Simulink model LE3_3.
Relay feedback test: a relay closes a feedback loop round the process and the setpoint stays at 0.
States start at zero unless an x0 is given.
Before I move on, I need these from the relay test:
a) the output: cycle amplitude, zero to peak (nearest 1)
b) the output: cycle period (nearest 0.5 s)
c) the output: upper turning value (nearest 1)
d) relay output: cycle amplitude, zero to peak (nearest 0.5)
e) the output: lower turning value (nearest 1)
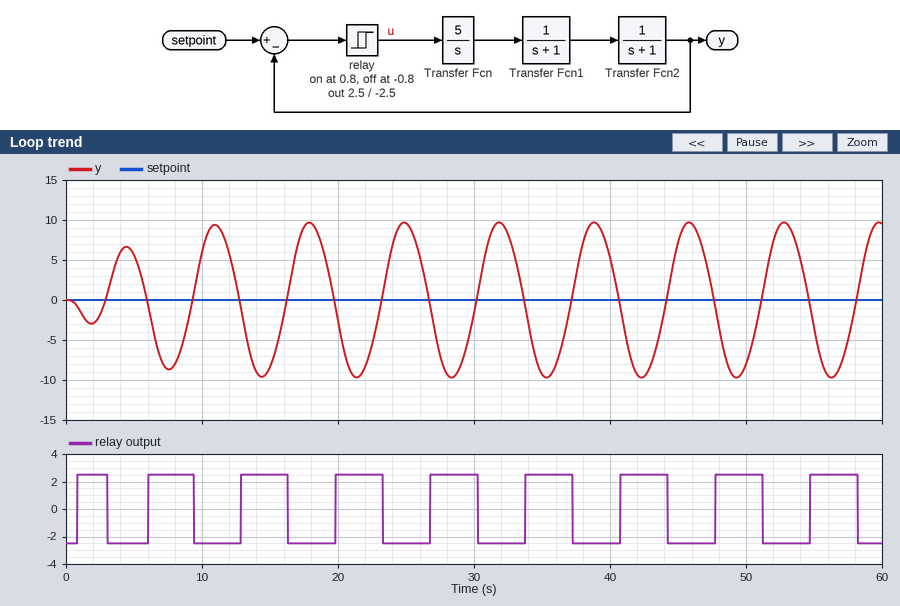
10
7.0 s
10
2.5
-10
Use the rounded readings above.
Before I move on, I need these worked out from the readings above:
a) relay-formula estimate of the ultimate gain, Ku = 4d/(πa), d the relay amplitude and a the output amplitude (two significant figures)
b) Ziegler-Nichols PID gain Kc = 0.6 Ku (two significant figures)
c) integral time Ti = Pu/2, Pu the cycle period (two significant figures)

0.32
0.19
3.5 s
